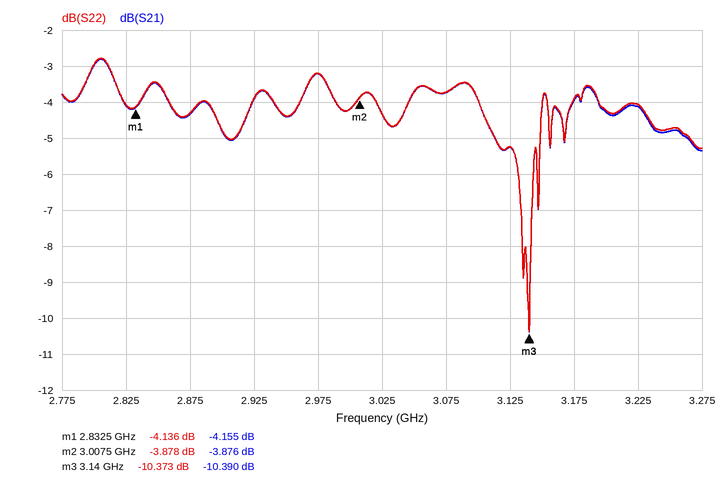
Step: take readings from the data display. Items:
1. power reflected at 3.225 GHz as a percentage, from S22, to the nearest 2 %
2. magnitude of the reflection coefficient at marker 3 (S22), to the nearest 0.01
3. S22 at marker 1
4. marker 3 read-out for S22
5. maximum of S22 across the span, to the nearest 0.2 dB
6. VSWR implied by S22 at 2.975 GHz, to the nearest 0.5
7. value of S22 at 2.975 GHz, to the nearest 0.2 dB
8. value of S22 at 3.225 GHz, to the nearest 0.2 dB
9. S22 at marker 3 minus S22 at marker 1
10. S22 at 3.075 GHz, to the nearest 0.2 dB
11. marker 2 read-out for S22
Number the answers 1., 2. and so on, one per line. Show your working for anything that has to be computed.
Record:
1. 10^(-4/10) ≈ 40 %
2. 10^(-10.373/20) ≈ 0.30
3. -4.136 dB
4. -10.373 dB
5. -2.8 dB
6. |Γ| = 10^(-3.2/20) = 0.6918; VSWR = (1 + 0.6918)/(1 − 0.6918) ≈ 5.5
7. -3.2 dB
8. -4.0 dB
9. -10.373 − (-4.136) = -6.237 dB
10. -3.8 dB
11. -3.878 dB
